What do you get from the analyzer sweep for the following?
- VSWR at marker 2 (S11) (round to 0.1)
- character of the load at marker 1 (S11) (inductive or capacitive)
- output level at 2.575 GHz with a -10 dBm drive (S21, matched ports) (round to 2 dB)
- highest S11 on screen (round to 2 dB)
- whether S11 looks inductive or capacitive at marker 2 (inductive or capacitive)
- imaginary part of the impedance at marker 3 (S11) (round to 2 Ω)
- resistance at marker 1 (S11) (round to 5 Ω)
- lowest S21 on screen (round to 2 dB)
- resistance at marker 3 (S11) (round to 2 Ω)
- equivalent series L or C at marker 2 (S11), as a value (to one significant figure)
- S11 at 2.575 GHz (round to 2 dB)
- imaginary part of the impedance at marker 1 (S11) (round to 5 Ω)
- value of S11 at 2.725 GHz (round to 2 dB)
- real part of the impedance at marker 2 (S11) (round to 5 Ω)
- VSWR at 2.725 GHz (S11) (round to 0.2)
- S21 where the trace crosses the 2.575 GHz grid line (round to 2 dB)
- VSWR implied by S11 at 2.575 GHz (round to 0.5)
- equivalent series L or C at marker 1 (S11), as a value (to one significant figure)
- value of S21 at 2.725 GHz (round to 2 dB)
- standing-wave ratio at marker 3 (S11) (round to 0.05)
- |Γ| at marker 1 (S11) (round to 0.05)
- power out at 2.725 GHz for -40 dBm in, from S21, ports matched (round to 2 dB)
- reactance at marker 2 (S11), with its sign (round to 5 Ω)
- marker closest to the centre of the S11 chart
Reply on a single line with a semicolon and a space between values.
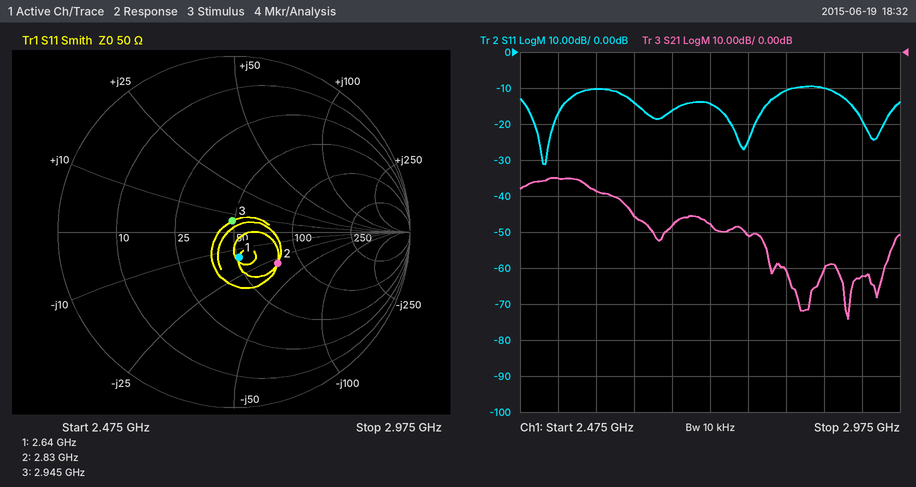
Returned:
1.9; capacitive; -48 dBm; -10 dB; capacitive; +6 Ω; 50 Ω; -74 dB; 48 Ω; 2 pF; -10 dB; -15 Ω; -14 dB; 75 Ω; 1.4; -38 dB; 2.0; 4 pF; -48 dB; 1.15; 0.15; -88 dBm; -30 Ω; marker 3
